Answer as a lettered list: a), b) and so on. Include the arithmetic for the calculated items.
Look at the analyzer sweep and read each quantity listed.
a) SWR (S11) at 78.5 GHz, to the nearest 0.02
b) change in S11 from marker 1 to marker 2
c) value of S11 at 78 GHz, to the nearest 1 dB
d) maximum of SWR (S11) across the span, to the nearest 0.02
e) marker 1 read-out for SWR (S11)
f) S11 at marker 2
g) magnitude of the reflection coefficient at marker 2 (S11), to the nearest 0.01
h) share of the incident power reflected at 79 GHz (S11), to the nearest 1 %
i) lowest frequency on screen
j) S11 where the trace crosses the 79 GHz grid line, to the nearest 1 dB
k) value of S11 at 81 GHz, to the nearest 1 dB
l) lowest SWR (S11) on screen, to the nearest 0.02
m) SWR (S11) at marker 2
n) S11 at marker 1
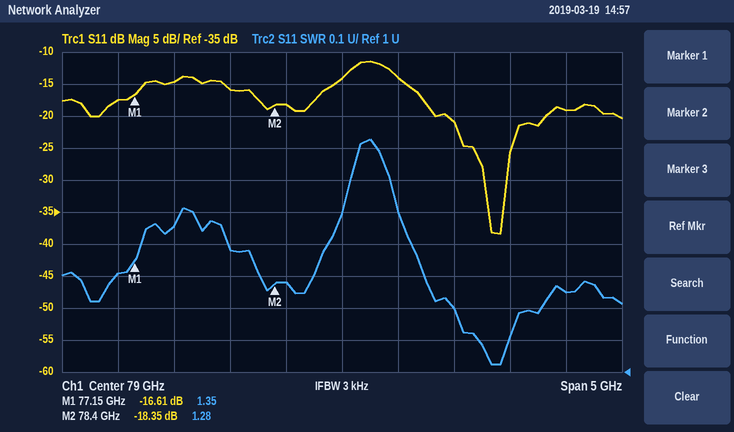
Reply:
a) 1.28
b) -18.35 − (-16.61) = -1.74 dB
c) -16 dB
d) 1.72
e) 1.35
f) -18.35 dB
g) 10^(-18.35/20) ≈ 0.12
h) 10^(-14/10) ≈ 4 %
i) 76.5 GHz
j) -14 dB
k) -19 dB
l) 1.02
m) 1.28
n) -16.61 dB
